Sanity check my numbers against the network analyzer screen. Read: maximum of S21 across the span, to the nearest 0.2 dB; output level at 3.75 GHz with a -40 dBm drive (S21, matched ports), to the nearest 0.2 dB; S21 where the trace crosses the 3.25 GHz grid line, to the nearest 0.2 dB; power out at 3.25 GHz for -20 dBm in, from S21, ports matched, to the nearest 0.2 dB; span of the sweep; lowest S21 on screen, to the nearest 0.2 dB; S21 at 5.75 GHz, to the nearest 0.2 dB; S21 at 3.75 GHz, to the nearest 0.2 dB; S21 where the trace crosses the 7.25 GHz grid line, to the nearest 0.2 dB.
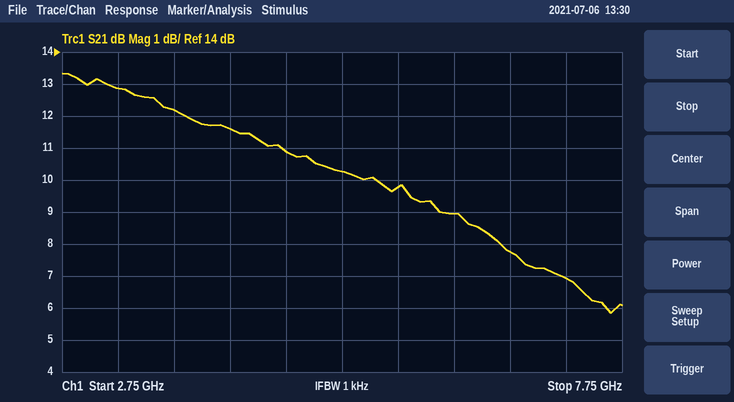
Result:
13.4 dB
-27.8 dBm
12.8 dB
-7.2 dBm
5 GHz
5.8 dB
9.8 dB
12.2 dB
7.0 dB
